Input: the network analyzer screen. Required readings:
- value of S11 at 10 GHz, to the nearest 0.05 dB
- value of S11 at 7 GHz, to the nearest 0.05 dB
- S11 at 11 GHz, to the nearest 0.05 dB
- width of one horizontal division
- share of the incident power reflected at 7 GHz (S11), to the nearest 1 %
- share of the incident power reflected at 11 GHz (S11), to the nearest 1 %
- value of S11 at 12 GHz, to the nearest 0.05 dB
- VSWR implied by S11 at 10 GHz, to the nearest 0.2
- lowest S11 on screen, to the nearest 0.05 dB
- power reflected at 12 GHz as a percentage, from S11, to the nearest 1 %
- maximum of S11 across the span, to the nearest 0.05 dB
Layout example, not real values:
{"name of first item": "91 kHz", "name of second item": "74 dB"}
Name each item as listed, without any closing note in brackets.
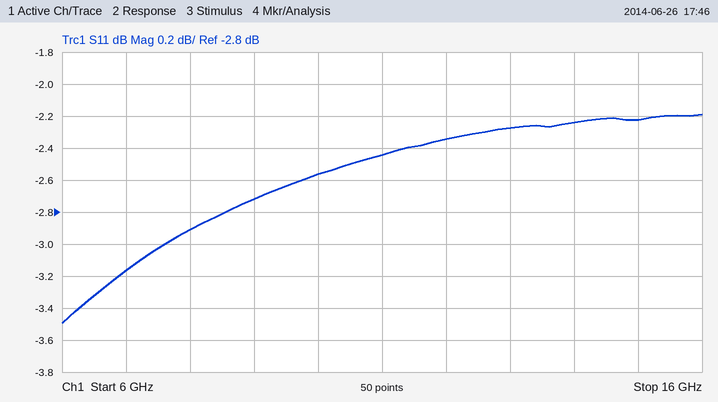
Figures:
{"value of S11 at 10 GHz, to the nearest 0.05 dB": "-2.55 dB", "value of S11 at 7 GHz, to the nearest 0.05 dB": "-3.15 dB", "S11 at 11 GHz, to the nearest 0.05 dB": "-2.45 dB", "width of one horizontal division": "1 GHz", "share of the incident power reflected at 7 GHz (S11), to the nearest 1 %": "48 %", "share of the incident power reflected at 11 GHz (S11), to the nearest 1 %": "57 %", "value of S11 at 12 GHz, to the nearest 0.05 dB": "-2.35 dB", "VSWR implied by S11 at 10 GHz, to the nearest 0.2": "6.8", "lowest S11 on screen, to the nearest 0.05 dB": "-3.50 dB", "power reflected at 12 GHz as a percentage, from S11, to the nearest 1 %": "58 %", "maximum of S11 across the span, to the nearest 0.05 dB": "-2.20 dB"}
